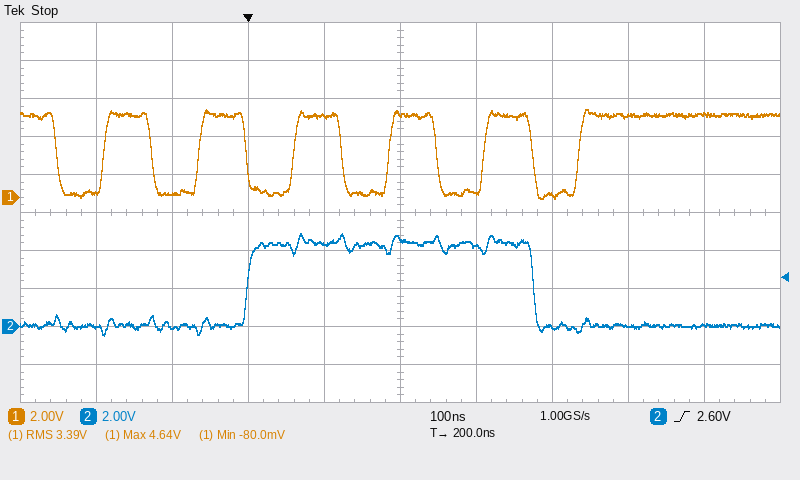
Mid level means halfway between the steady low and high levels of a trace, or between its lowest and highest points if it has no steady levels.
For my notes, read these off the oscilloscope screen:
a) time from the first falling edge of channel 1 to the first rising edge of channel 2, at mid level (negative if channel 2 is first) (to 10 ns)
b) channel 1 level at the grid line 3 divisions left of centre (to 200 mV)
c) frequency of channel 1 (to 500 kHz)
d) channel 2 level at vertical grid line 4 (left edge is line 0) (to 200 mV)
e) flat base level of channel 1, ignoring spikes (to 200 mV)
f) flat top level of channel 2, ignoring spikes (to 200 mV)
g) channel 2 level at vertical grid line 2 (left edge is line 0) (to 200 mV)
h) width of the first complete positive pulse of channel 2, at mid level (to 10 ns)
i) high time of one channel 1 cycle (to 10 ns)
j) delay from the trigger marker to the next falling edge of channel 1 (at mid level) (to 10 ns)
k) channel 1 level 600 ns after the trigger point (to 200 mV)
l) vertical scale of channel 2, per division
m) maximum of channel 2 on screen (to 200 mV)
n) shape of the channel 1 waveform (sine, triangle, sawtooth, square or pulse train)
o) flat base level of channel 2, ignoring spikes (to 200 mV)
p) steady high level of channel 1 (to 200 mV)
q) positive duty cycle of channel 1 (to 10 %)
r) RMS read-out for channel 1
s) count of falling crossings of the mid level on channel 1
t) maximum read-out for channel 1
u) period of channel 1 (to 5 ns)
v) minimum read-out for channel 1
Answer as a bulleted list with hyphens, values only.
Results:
- +250 ns
- 200 mV
- 8.0 MHz
- 4.4 V
- 200 mV
- 4.4 V
- 0.0 V
- 380 ns
- 60 ns
- 120 ns
- 4.4 V
- 2 V
- 4.8 V
- square
- 0.0 V
- 4.4 V
- 50 %
- 3.39 V
- 6
- 4.64 V
- 125 ns
- -80.0 mV
